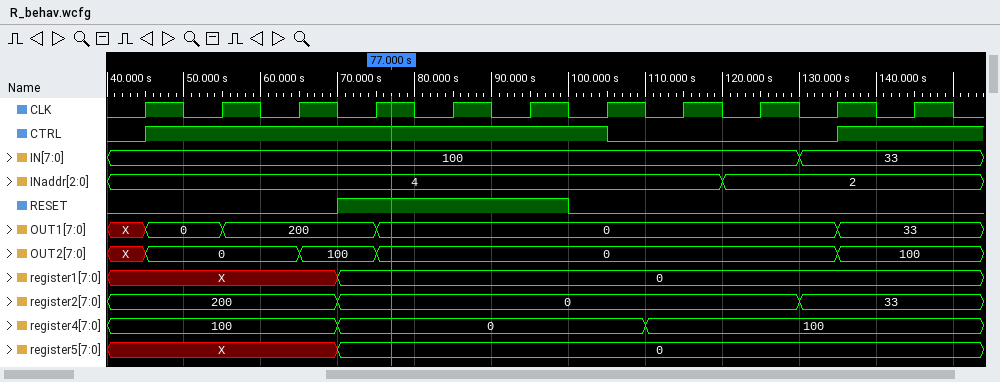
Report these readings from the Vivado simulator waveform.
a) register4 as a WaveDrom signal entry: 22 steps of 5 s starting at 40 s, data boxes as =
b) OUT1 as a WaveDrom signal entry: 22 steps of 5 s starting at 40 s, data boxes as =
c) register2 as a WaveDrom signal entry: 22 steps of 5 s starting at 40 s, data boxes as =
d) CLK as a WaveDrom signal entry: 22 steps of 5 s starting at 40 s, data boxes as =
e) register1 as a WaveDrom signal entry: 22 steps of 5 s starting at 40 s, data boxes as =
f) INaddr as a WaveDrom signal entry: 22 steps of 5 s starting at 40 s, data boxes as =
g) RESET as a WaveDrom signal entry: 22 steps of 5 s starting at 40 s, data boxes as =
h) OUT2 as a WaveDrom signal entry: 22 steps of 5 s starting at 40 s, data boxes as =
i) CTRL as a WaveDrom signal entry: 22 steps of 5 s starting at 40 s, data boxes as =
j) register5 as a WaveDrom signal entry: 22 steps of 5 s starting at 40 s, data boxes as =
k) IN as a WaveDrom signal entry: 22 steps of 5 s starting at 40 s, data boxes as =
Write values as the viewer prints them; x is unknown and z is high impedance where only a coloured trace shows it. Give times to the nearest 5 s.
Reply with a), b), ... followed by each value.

a) {name: 'register4', wave: '=.....=.......=.......', data: '100 0 100'}
b) {name: 'OUT1', wave: 'x=.=...=...........=..', data: '0 200 0 33'}
c) {name: 'register2', wave: '=.....=...........=...', data: '200 0 33'}
d) {name: 'CLK', wave: '0101010101010101010101'}
e) {name: 'register1', wave: 'x.....=...............', data: '0'}
f) {name: 'INaddr', wave: '=...............=.....', data: '4 2'}
g) {name: 'RESET', wave: '0.....1.....0.........'}
h) {name: 'OUT2', wave: 'x=...=.=...........=..', data: '0 100 0 100'}
i) {name: 'CTRL', wave: '01...........0.....1..'}
j) {name: 'register5', wave: 'x.....=...............', data: '0'}
k) {name: 'IN', wave: '=.................=...', data: '100 33'}
